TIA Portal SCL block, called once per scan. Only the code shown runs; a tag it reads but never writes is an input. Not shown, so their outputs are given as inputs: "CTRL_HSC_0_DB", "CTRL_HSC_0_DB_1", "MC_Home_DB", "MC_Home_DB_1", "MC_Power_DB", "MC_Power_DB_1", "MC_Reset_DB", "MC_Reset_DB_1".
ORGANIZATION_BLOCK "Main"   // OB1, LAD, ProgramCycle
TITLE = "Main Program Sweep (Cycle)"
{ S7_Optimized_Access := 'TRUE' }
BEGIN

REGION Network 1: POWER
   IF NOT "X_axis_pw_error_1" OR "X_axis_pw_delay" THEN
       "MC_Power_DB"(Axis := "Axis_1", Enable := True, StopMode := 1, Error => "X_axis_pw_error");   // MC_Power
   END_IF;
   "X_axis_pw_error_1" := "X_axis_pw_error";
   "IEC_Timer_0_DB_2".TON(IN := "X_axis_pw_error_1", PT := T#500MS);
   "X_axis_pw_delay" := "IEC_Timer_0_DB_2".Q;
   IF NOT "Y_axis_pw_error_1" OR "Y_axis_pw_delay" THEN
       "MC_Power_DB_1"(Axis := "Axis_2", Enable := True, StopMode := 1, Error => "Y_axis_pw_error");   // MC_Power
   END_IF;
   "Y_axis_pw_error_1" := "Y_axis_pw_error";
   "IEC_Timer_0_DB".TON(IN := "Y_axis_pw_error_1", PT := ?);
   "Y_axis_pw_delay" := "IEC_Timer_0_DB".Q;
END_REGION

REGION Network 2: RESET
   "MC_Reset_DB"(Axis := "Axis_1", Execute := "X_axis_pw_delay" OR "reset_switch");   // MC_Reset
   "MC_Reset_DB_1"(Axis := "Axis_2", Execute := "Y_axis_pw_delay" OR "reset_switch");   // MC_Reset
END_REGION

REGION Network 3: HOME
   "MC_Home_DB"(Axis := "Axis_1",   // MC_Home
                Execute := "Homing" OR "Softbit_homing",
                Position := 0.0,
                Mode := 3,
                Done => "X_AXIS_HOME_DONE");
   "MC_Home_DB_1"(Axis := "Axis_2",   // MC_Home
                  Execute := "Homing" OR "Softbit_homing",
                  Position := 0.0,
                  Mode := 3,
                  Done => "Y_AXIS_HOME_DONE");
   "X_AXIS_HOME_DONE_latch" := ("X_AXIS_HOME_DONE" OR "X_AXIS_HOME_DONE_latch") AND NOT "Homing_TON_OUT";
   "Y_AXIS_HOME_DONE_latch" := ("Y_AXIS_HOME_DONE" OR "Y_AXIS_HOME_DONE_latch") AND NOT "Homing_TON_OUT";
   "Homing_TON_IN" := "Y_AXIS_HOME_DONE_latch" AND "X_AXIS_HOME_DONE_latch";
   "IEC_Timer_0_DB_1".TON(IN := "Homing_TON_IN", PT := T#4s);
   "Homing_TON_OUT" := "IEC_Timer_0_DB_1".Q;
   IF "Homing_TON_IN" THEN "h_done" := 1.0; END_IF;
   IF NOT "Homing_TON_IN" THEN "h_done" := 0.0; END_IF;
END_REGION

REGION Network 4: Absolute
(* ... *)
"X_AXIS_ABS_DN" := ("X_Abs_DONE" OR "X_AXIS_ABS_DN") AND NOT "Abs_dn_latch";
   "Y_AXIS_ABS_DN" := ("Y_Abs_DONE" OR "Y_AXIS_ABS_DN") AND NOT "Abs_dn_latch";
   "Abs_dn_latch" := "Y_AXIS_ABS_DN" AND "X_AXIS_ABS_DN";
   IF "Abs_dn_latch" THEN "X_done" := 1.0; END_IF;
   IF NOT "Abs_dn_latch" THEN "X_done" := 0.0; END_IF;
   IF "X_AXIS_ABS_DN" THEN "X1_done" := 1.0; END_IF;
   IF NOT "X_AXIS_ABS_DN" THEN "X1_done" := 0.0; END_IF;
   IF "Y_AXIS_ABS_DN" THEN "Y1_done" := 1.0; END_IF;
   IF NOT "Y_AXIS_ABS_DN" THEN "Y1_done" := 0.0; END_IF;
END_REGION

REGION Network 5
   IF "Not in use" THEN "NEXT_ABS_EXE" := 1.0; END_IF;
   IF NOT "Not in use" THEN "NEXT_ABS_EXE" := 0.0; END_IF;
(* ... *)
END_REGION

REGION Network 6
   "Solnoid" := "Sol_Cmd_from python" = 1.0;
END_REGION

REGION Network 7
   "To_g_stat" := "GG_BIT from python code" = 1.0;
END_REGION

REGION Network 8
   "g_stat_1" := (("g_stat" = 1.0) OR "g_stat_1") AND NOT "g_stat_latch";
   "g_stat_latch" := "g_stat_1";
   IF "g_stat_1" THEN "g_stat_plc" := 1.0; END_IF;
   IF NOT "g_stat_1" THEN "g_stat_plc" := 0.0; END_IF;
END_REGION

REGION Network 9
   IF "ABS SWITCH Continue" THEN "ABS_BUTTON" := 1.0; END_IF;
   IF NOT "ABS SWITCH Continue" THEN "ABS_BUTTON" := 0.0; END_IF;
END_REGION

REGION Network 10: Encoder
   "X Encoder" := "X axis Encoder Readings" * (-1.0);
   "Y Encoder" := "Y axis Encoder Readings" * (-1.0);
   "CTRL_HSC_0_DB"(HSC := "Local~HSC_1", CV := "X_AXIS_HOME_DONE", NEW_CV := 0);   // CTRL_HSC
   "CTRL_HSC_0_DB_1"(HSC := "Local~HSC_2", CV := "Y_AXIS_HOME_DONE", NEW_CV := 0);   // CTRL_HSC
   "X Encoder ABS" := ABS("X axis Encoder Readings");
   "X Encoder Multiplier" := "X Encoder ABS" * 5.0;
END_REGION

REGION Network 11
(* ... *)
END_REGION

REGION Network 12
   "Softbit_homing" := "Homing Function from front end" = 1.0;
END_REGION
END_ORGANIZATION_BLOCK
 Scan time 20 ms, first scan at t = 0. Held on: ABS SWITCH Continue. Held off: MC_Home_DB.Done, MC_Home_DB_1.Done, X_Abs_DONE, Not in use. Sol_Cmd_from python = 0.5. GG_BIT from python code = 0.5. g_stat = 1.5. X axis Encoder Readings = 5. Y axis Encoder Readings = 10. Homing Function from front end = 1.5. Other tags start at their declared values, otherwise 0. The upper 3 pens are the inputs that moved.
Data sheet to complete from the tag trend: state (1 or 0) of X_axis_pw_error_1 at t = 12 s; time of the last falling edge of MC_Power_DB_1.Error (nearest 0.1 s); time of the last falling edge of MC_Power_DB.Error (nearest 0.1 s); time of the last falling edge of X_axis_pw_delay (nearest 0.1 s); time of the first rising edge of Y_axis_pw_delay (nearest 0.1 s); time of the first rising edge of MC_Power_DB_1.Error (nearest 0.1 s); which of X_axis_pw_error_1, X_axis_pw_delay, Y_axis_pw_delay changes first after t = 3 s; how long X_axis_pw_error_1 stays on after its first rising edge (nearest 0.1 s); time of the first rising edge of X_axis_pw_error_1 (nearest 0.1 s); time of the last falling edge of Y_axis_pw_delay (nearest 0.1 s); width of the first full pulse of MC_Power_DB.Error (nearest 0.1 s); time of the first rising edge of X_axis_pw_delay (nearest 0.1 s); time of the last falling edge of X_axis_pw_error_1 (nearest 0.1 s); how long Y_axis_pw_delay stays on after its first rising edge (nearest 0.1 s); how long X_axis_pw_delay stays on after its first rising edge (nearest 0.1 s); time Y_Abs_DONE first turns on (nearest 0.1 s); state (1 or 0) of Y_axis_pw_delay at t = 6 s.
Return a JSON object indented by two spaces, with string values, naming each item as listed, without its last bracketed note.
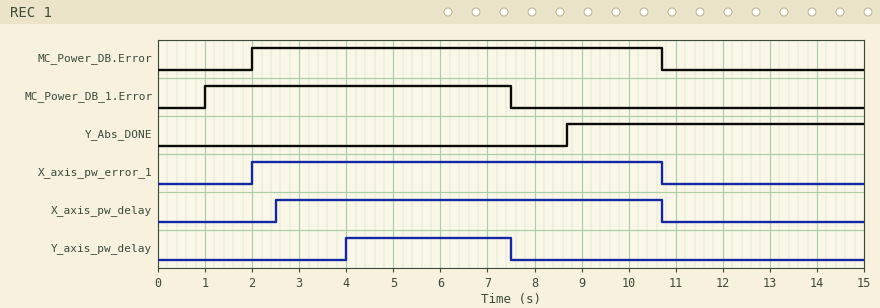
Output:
{
  "state (1 or 0) of X_axis_pw_error_1 at t = 12 s": "0",
  "time of the last falling edge of MC_Power_DB_1.Error": "7.5 s",
  "time of the last falling edge of MC_Power_DB.Error": "10.7 s",
  "time of the last falling edge of X_axis_pw_delay": "10.7 s",
  "time of the first rising edge of Y_axis_pw_delay": "4.0 s",
  "time of the first rising edge of MC_Power_DB_1.Error": "1.0 s",
  "which of X_axis_pw_error_1, X_axis_pw_delay, Y_axis_pw_delay changes first after t = 3 s": "Y_axis_pw_delay",
  "how long X_axis_pw_error_1 stays on after its first rising edge": "8.7 s",
  "time of the first rising edge of X_axis_pw_error_1": "2.0 s",
  "time of the last falling edge of Y_axis_pw_delay": "7.5 s",
  "width of the first full pulse of MC_Power_DB.Error": "8.7 s",
  "time of the first rising edge of X_axis_pw_delay": "2.5 s",
  "time of the last falling edge of X_axis_pw_error_1": "10.7 s",
  "how long Y_axis_pw_delay stays on after its first rising edge": "3.5 s",
  "how long X_axis_pw_delay stays on after its first rising edge": "8.2 s",
  "time Y_Abs_DONE first turns on": "8.7 s",
  "state (1 or 0) of Y_axis_pw_delay at t = 6 s": "1"
}
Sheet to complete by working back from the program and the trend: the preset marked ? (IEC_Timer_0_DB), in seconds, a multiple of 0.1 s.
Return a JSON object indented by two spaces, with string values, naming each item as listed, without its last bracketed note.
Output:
{
  "the preset marked ? (IEC_Timer_0_DB), in seconds, a multiple of 0.1 s": "3.0 s"
}
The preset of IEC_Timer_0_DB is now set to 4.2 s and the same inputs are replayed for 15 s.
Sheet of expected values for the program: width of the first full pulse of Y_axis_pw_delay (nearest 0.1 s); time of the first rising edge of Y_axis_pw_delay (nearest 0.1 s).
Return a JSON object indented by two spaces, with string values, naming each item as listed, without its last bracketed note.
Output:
{
  "width of the first full pulse of Y_axis_pw_delay": "2.3 s",
  "time of the first rising edge of Y_axis_pw_delay": "5.2 s"
}
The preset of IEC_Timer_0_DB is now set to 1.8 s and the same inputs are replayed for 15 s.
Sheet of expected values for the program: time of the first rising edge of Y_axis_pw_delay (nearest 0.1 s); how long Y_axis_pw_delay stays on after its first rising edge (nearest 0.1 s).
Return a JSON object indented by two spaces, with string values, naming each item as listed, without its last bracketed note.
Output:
{
  "time of the first rising edge of Y_axis_pw_delay": "2.8 s",
  "how long Y_axis_pw_delay stays on after its first rising edge": "4.7 s"
}
